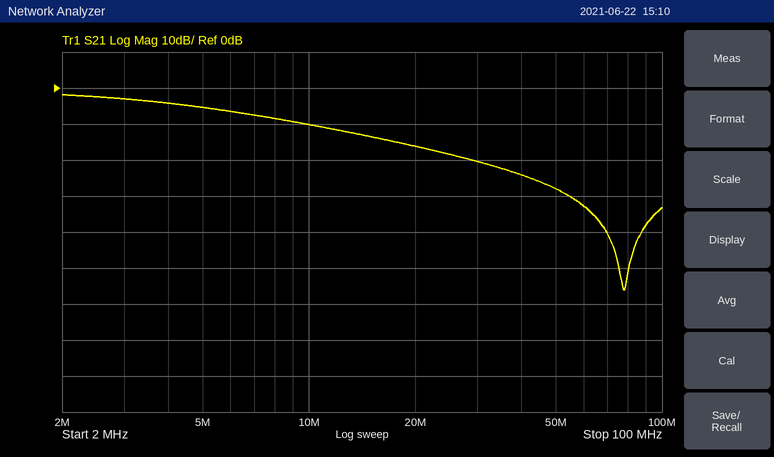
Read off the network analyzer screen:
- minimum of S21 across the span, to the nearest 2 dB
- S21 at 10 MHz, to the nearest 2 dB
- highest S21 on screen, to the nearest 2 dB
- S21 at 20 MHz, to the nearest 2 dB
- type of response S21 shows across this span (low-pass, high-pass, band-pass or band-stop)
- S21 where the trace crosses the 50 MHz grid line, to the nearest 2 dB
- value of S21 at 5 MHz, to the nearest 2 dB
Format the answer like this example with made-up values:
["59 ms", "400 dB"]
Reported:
["-56 dB", "-10 dB", "-2 dB", "-16 dB", "low-pass", "-28 dB", "-6 dB"]
